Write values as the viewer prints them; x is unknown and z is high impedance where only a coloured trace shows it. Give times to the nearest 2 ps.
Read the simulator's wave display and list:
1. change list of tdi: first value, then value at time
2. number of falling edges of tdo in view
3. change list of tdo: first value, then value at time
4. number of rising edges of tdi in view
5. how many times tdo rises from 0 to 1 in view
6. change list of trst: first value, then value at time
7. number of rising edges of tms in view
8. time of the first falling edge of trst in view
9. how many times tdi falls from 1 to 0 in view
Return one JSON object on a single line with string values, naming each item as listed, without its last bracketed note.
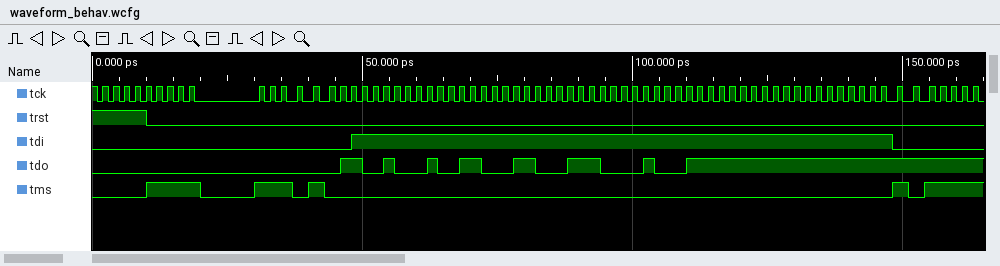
{"change list of tdi: first value, then value at time": "0, 1 at 48 ps, 0 at 148 ps", "number of falling edges of tdo in view": "7", "change list of tdo: first value, then value at time": "0, 1 at 46 ps, 0 at 50 ps, 1 at 54 ps, 0 at 56 ps, 1 at 62 ps, 0 at 64 ps, 1 at 68 ps, 0 at 72 ps, 1 at 78 ps, 0 at 82 ps, 1 at 88 ps, 0 at 94 ps, 1 at 102 ps, 0 at 104 ps, 1 at 110 ps", "number of rising edges of tdi in view": "1", "how many times tdo rises from 0 to 1 in view": "8", "change list of trst: first value, then value at time": "1, 0 at 10 ps", "number of rising edges of tms in view": "5", "time of the first falling edge of trst in view": "10 ps", "how many times tdi falls from 1 to 0 in view": "1"}
